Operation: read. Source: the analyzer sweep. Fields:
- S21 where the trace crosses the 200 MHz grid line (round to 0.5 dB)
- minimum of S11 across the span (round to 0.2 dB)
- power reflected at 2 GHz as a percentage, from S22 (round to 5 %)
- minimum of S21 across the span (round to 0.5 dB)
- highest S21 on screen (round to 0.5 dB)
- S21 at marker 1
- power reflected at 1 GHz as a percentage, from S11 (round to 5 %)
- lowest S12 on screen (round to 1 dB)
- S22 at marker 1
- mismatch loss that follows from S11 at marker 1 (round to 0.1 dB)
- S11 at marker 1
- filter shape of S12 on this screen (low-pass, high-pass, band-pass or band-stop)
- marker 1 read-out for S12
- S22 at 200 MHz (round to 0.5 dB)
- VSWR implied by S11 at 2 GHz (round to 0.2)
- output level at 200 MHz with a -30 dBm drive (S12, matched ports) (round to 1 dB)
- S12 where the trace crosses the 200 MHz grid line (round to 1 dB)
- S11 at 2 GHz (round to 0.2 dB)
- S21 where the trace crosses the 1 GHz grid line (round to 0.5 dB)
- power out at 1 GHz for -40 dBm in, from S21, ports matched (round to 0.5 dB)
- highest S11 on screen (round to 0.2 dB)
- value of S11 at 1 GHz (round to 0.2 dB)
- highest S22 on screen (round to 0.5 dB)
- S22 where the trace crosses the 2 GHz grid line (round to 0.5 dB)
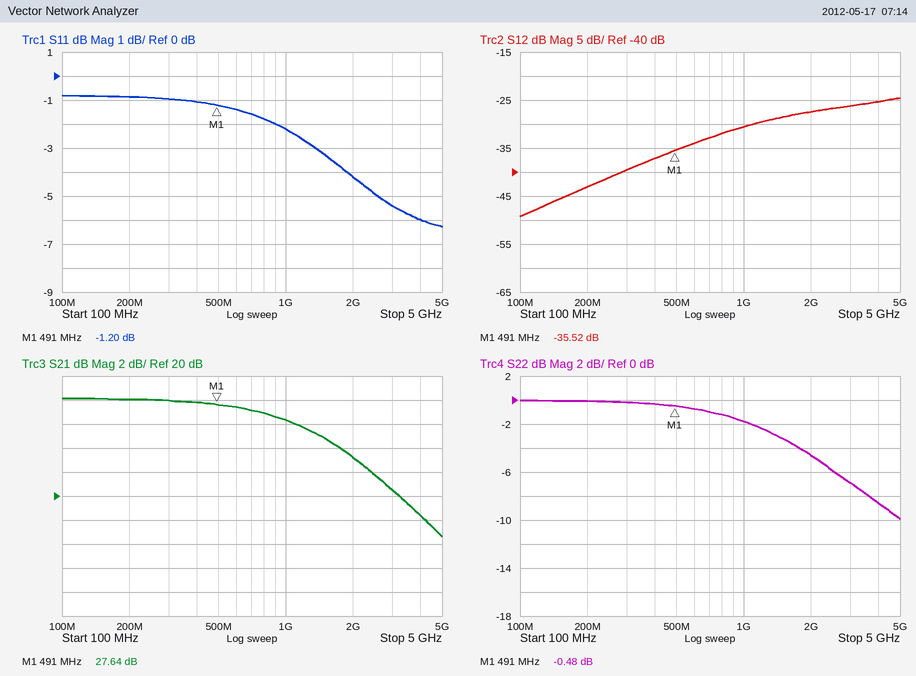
28.0 dB
-6.2 dB
35 %
16.5 dB
28.0 dB
27.64 dB
60 %
-49 dB
-0.48 dB
6.2 dB
-1.20 dB
high-pass
-35.52 dB
0.0 dB
4.2
-73 dBm
-43 dB
-4.2 dB
26.5 dB
-13.5 dBm
-0.8 dB
-2.2 dB
0.0 dB
-4.5 dB
